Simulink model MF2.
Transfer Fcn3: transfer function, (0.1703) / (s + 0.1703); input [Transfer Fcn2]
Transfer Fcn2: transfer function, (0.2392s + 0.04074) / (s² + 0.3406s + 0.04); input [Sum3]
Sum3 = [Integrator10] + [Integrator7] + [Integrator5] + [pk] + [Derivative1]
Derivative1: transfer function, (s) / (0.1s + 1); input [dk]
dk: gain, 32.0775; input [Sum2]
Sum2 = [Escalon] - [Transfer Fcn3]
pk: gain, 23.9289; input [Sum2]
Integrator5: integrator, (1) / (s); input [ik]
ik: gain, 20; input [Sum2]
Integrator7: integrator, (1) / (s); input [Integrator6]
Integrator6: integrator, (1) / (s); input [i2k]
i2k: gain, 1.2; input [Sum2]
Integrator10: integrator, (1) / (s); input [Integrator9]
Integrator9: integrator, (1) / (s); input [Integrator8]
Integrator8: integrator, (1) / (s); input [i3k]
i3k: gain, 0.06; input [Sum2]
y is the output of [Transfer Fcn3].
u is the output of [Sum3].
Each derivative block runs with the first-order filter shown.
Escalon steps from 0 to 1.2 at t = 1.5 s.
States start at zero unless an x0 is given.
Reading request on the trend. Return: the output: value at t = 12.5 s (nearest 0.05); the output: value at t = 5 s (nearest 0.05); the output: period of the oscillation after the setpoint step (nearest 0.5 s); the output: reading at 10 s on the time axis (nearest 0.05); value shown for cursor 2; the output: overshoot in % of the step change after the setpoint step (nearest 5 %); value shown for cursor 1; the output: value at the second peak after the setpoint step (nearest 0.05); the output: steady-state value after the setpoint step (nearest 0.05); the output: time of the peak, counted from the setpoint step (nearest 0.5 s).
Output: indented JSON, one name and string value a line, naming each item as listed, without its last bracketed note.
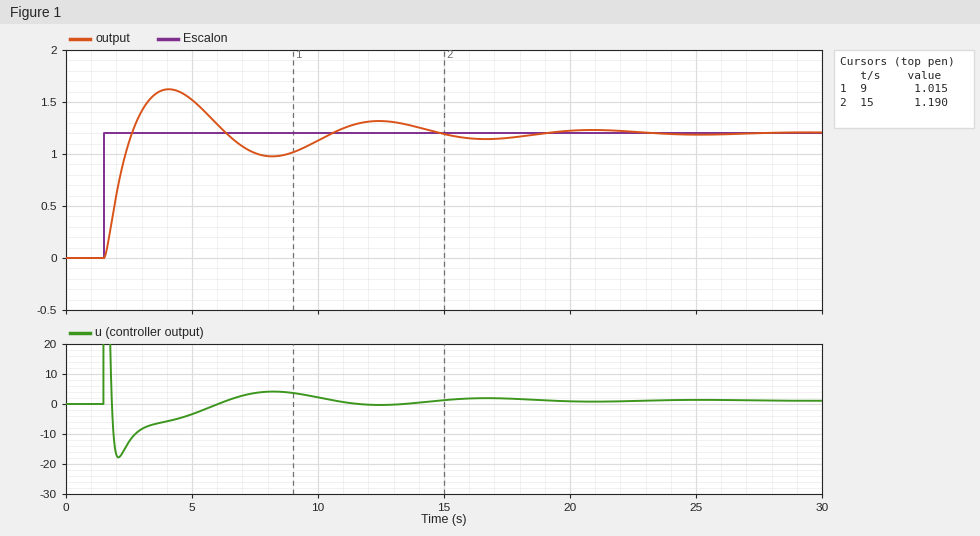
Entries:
{
  "the output: value at t = 12.5 s": "1.30",
  "the output: value at t = 5 s": "1.50",
  "the output: period of the oscillation after the setpoint step": "8.5 s",
  "the output: reading at 10 s on the time axis": "1.15",
  "value shown for cursor 2": "1.190",
  "the output: overshoot in % of the step change after the setpoint step": "35 %",
  "value shown for cursor 1": "1.015",
  "the output: value at the second peak after the setpoint step": "1.30",
  "the output: steady-state value after the setpoint step": "1.20",
  "the output: time of the peak, counted from the setpoint step": "2.5 s"
}
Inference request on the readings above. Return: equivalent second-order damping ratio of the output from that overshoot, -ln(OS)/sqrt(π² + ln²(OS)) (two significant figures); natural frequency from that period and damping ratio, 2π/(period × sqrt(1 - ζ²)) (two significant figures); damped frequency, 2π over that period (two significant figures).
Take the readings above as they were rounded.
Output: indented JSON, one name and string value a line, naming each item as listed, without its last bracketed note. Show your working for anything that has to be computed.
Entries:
{
  "equivalent second-order damping ratio of the output from that overshoot, -ln(OS)/sqrt(π² + ln²(OS))": "ln(0.35) = -1.050; 1.050 / sqrt(9.870 + 1.102) = 0.32",
  "natural frequency from that period and damping ratio, 2π/(period × sqrt(1 - ζ²))": "2π / (8.5 × sqrt(1 - 0.32²)) = 0.78 rad/s",
  "damped frequency, 2π over that period": "2π / 8.5 = 0.74 rad/s"
}
